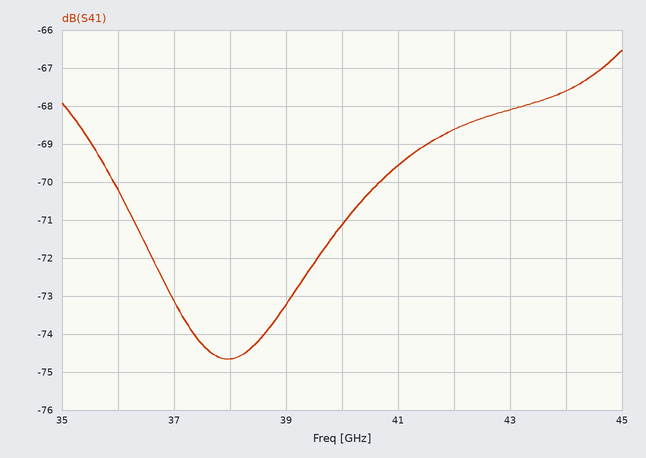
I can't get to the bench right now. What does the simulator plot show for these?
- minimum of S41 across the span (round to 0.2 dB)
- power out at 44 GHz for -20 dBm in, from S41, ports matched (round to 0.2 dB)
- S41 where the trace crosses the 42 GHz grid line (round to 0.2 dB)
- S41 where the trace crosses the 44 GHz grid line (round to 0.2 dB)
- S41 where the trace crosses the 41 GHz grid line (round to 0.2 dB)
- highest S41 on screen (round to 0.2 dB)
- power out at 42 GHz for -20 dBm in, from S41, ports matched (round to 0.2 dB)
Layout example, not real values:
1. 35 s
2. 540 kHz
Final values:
1. -74.6 dB
2. -87.6 dBm
3. -68.6 dB
4. -67.6 dB
5. -69.6 dB
6. -66.6 dB
7. -88.6 dBm
